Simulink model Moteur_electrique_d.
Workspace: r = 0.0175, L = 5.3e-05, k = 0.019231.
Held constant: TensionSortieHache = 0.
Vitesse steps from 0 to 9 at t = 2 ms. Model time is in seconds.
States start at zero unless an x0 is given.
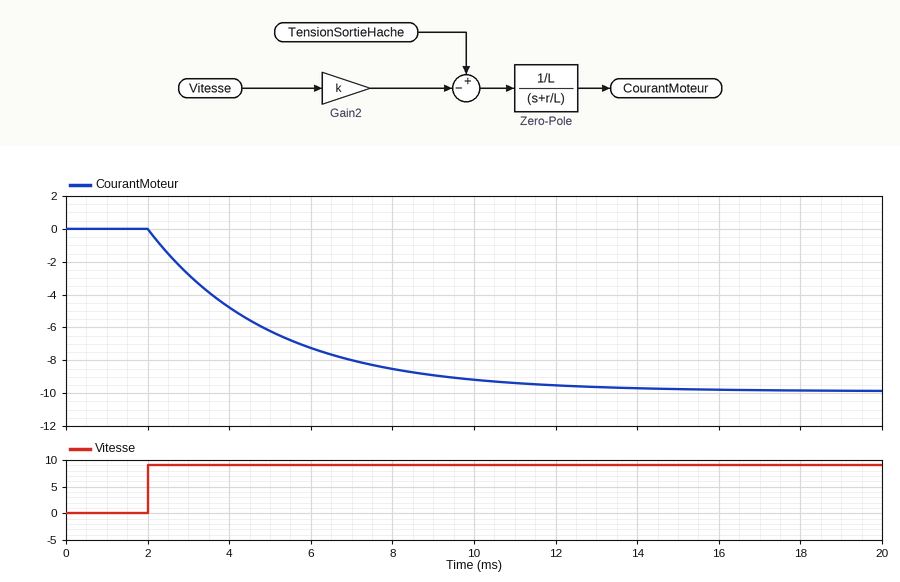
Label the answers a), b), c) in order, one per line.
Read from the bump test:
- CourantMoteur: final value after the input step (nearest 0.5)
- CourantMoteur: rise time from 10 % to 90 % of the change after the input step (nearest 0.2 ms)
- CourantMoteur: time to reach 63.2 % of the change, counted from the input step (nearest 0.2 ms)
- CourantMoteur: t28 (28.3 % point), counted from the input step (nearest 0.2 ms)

a) -10.0
b) 6.6 ms
c) 3.0 ms
d) 1.0 ms
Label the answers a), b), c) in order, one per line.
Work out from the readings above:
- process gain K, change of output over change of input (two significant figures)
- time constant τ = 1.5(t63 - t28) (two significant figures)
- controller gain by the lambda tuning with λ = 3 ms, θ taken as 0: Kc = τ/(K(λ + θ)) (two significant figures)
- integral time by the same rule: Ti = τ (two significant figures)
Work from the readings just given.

a) -1.1
b) 3.0 ms
c) -0.91
d) 3.0 ms
